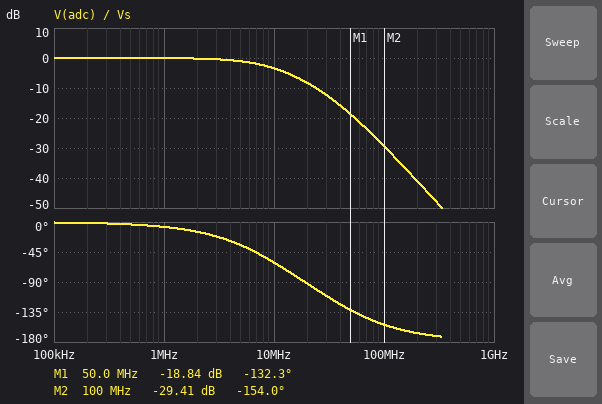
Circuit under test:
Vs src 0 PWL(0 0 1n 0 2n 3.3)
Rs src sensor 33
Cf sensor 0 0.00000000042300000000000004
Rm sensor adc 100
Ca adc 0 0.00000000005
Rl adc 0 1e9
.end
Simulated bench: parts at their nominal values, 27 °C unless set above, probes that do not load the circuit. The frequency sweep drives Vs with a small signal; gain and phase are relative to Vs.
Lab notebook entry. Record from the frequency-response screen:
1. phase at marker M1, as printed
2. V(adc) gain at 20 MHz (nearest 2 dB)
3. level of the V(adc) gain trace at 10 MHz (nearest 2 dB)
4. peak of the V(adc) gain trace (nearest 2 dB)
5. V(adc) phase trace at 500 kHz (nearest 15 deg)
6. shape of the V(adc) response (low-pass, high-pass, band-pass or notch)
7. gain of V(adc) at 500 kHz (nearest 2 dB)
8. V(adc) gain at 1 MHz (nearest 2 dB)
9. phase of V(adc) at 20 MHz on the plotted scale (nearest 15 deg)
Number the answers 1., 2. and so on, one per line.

1. -132.3 deg
2. -8 dB
3. -4 dB
4. 0 dB
5. 0 deg
6. low-pass
7. 0 dB
8. 0 dB
9. -90 deg
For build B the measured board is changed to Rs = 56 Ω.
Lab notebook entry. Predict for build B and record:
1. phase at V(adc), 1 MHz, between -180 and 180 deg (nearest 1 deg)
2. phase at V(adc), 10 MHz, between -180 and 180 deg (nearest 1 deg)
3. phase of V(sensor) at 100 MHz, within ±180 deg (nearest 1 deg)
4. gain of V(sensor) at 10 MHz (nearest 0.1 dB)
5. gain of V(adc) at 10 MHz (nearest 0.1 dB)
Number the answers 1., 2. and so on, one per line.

1. -11 deg
2. -75 deg
3. -84 deg
4. -5.8 dB
5. -6.2 dB
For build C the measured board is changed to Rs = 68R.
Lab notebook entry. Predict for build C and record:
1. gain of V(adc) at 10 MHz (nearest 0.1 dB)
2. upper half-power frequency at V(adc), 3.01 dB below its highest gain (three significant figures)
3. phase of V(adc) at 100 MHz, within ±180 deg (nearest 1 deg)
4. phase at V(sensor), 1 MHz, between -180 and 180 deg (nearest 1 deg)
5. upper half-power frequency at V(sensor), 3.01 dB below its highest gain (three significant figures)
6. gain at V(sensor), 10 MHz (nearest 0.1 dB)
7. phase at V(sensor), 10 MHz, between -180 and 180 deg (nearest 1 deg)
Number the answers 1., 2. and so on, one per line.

1. -7.5 dB
2. 4.77 MHz
3. -157 deg
4. -11 deg
5. 4.88 MHz
6. -7.1 dB
7. -62 deg
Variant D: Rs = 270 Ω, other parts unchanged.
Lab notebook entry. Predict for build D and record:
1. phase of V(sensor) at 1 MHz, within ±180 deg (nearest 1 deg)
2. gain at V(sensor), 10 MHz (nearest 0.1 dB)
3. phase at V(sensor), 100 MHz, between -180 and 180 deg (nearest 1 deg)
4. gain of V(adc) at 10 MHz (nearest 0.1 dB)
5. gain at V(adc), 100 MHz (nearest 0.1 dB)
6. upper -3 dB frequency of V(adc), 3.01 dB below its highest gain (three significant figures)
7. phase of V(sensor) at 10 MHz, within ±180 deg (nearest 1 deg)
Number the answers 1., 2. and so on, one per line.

1. -39 deg
2. -18.1 dB
3. -87 deg
4. -18.5 dB
5. -47.6 dB
6. 1.24 MHz
7. -81 deg
